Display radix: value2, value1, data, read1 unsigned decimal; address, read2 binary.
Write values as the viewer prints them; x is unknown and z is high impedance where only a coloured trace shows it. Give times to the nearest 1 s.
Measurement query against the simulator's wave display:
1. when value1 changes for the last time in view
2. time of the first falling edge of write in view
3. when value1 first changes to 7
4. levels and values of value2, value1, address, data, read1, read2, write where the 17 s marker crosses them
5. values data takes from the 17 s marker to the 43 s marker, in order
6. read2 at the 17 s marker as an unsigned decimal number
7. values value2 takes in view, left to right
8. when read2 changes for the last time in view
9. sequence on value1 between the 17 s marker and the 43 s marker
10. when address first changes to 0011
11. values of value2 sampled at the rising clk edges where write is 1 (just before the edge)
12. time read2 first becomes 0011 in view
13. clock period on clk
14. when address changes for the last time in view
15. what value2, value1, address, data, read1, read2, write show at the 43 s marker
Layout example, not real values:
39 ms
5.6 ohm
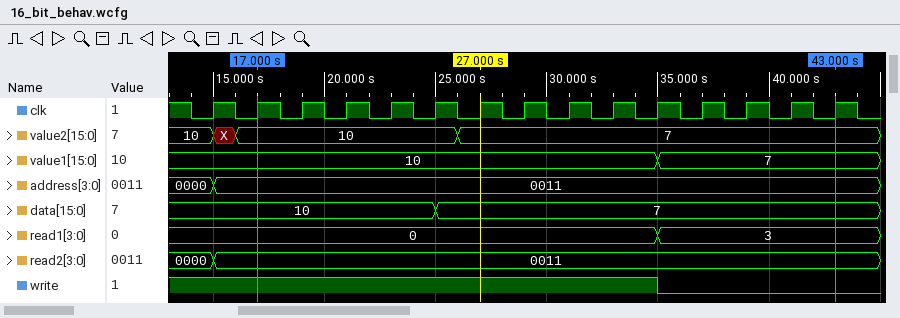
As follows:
35 s
35 s
35 s
value2=10, value1=10, address=0011, data=10, read1=0, read2=0011, write=1
10, 7
3
10, X, 10, 7
15 s
10, 7
15 s
10, 10, 10, 10, 10, 10, 7, 7, 7, 7, 7
15 s
2 s
15 s
value2=7, value1=7, address=0011, data=7, read1=3, read2=0011, write=0
